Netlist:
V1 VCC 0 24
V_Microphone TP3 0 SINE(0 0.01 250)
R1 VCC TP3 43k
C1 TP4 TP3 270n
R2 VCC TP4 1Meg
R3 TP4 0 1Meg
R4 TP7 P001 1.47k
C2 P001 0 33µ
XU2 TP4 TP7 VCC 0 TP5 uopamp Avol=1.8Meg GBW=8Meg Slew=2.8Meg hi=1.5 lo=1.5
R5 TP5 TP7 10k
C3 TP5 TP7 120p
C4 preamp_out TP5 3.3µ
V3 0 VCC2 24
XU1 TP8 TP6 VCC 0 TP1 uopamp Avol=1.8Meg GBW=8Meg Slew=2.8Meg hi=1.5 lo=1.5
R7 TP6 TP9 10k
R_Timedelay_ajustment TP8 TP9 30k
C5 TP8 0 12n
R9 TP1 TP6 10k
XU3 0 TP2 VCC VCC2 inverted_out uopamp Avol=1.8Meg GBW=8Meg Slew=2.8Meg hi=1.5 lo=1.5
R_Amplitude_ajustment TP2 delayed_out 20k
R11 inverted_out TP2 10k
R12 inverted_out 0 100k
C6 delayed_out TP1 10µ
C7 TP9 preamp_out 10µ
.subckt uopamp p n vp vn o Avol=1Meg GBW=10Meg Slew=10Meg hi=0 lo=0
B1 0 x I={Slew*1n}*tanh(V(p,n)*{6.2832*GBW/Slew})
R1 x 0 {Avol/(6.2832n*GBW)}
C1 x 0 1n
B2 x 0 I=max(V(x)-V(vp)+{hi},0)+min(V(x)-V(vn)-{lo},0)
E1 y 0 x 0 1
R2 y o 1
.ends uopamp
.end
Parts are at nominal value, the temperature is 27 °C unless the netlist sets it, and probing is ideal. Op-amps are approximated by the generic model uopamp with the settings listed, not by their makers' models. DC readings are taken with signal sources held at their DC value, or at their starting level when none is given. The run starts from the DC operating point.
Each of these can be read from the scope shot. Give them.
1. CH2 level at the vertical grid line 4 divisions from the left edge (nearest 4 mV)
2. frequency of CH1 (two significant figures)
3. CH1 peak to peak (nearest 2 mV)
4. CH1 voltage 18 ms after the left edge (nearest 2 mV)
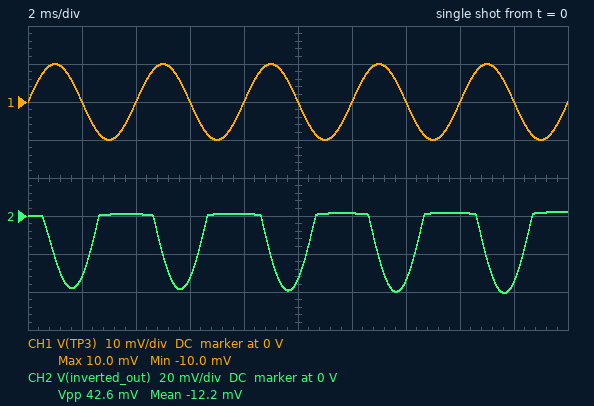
0 V
250 Hz
20 mV
0 V
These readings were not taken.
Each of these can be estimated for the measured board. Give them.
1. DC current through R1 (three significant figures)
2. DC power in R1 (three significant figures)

558 µA
13.4 mW
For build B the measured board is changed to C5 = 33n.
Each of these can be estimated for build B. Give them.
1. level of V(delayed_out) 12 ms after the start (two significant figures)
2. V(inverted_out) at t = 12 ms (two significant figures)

-3.0 mV
1.5 mV
